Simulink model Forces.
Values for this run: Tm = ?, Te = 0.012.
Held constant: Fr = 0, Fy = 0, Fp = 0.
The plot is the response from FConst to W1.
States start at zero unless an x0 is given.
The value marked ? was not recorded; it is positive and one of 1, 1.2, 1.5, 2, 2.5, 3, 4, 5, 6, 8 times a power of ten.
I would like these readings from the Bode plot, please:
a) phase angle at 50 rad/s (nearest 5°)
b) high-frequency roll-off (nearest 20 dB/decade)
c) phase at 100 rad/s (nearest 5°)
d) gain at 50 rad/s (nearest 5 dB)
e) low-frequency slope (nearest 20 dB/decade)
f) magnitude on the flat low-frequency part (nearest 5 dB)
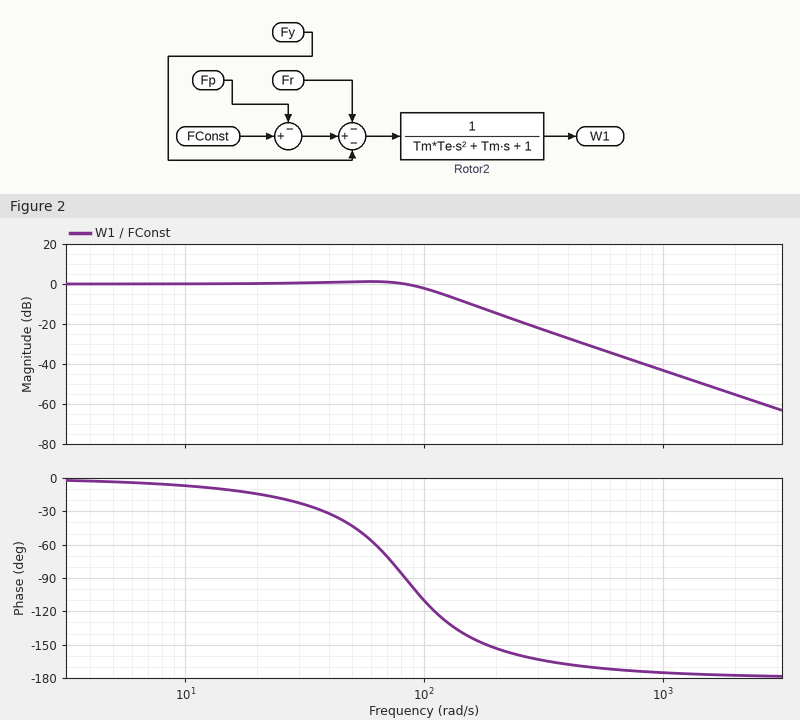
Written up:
-45°
-40 dB/decade
-110°
0 dB
0 dB/decade
0 dB
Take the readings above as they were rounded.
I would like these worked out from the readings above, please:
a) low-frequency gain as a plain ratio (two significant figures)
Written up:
1.0
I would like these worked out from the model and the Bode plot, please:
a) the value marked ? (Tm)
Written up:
0.012
